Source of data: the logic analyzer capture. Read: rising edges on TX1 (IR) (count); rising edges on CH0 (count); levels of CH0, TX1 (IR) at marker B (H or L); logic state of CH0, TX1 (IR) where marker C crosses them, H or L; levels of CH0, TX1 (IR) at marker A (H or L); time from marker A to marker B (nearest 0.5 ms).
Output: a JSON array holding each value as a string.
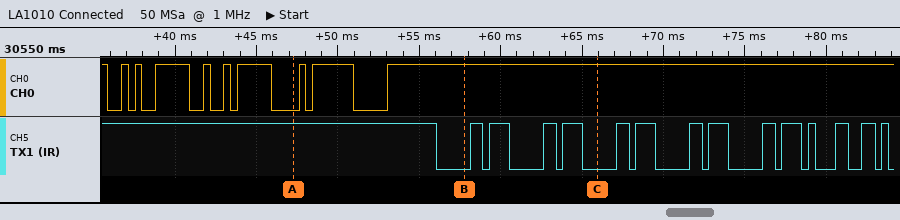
["14", "9", "CH0=H, TX1 (IR)=L", "CH0=H, TX1 (IR)=L", "CH0=L, TX1 (IR)=H", "10.5 ms"]
